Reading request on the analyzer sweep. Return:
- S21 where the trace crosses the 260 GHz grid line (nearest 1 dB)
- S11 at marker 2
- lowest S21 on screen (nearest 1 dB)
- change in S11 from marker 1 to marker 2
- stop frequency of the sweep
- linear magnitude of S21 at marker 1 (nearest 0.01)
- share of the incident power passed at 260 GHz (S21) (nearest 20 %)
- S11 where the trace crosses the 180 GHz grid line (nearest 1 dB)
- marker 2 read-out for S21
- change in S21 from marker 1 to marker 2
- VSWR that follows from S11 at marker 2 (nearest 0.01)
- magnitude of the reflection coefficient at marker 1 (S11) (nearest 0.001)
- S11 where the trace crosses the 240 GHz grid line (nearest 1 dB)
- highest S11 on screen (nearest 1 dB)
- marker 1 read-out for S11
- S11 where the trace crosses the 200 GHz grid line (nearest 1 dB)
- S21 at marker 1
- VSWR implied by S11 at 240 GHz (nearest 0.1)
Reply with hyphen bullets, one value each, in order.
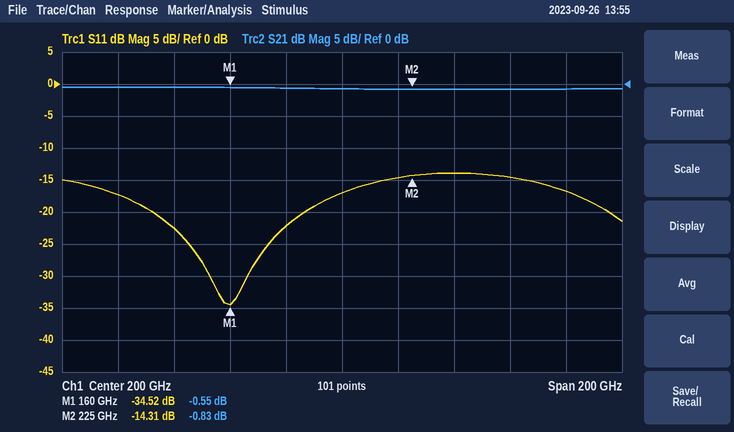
- -1 dB
- -14.31 dB
- -1 dB
- 20.21 dB
- 300 GHz
- 0.94
- 80 %
- -22 dB
- -0.83 dB
- -0.28 dB
- 1.48
- 0.019
- -14 dB
- -14 dB
- -34.52 dB
- -17 dB
- -0.55 dB
- 1.5
